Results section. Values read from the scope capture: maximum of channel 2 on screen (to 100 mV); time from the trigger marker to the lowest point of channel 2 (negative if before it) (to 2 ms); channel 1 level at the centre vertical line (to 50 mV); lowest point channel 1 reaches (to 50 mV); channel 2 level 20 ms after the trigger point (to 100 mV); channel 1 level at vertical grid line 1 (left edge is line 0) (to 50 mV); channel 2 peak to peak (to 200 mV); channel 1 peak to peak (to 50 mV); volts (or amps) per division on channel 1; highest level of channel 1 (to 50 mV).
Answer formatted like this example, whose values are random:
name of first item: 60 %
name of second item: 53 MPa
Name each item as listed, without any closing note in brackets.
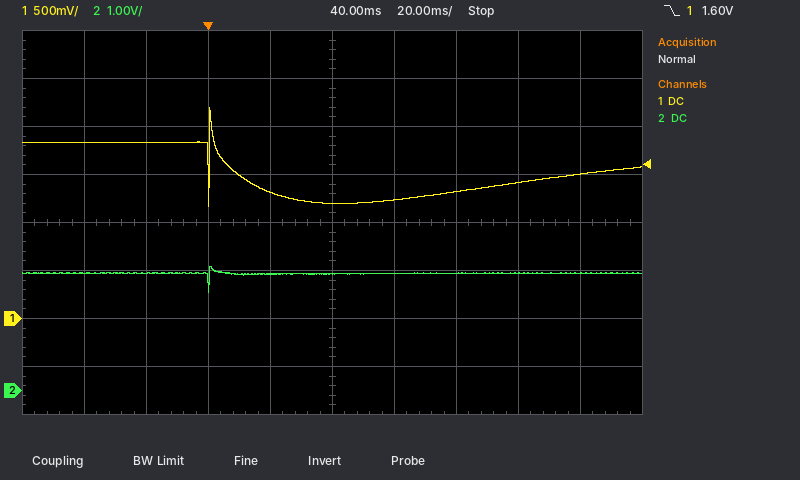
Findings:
maximum of channel 2 on screen: 2.6 V
time from the trigger marker to the lowest point of channel 2 (negative if before it): 0 ms
channel 1 level at the centre vertical line: 1.20 V
lowest point channel 1 reaches: 1.15 V
channel 2 level 20 ms after the trigger point: 2.4 V
channel 1 level at vertical grid line 1 (left edge is line 0): 1.85 V
channel 2 peak to peak: 600 mV
channel 1 peak to peak: 1.05 V
volts (or amps) per division on channel 1: 500 mV
highest level of channel 1: 2.20 V
